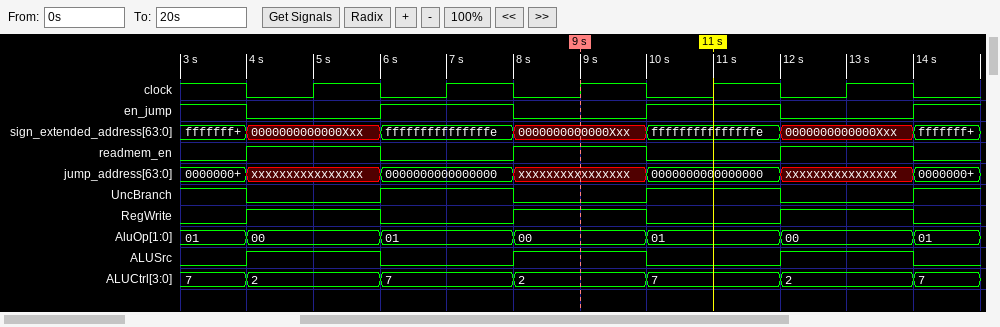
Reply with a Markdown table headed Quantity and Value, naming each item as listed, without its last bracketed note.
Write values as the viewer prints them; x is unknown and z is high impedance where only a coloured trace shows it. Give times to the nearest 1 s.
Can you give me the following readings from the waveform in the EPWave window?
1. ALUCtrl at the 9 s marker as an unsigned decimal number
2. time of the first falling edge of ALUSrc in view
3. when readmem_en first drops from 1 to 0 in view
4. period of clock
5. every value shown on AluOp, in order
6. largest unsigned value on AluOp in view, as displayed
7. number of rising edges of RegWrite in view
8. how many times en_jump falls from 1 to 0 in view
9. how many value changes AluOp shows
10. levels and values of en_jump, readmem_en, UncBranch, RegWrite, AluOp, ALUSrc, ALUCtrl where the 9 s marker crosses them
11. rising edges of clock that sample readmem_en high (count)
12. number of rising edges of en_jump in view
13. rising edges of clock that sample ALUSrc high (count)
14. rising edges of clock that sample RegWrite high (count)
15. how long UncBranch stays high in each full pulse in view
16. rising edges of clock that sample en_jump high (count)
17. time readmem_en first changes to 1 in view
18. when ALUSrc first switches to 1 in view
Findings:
| Quantity | Value |
|---|---|
| ALUCtrl at the 9 s marker as an unsigned decimal number | 2 |
| time of the first falling edge of ALUSrc in view | 6 s |
| when readmem_en first drops from 1 to 0 in view | 6 s |
| period of clock | 2 s |
| every value shown on AluOp, in order | 01, 00, 01, 00, 01, 00, 01 |
| largest unsigned value on AluOp in view, as displayed | 01 |
| number of rising edges of RegWrite in view | 3 |
| how many times en_jump falls from 1 to 0 in view | 3 |
| how many value changes AluOp shows | 6 |
| levels and values of en_jump, readmem_en, UncBranch, RegWrite, AluOp, ALUSrc, ALUCtrl where the 9 s marker crosses them | en_jump=0, readmem_en=1, UncBranch=0, RegWrite=1, AluOp=00, ALUSrc=1, ALUCtrl=2 |
| rising edges of clock that sample readmem_en high | 3 |
| number of rising edges of en_jump in view | 3 |
| rising edges of clock that sample ALUSrc high | 3 |
| rising edges of clock that sample RegWrite high | 3 |
| how long UncBranch stays high in each full pulse in view | 2 s, 2 s |
| rising edges of clock that sample en_jump high | 2 |
| time readmem_en first changes to 1 in view | 4 s |
| when ALUSrc first switches to 1 in view | 4 s |
